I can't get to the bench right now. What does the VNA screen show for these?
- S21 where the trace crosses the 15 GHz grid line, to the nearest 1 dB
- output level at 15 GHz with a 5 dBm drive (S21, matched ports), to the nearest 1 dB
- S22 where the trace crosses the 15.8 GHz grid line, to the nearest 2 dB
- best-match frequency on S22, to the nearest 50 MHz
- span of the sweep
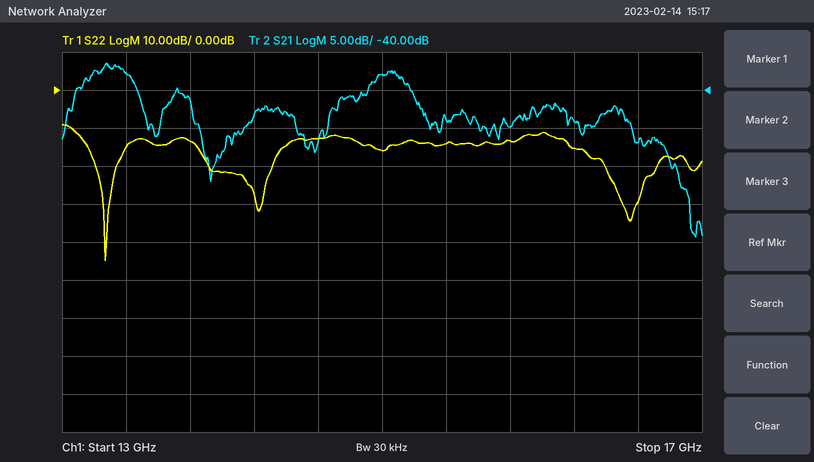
-38 dB
-33 dBm
-14 dB
13.25 GHz
4 GHz
